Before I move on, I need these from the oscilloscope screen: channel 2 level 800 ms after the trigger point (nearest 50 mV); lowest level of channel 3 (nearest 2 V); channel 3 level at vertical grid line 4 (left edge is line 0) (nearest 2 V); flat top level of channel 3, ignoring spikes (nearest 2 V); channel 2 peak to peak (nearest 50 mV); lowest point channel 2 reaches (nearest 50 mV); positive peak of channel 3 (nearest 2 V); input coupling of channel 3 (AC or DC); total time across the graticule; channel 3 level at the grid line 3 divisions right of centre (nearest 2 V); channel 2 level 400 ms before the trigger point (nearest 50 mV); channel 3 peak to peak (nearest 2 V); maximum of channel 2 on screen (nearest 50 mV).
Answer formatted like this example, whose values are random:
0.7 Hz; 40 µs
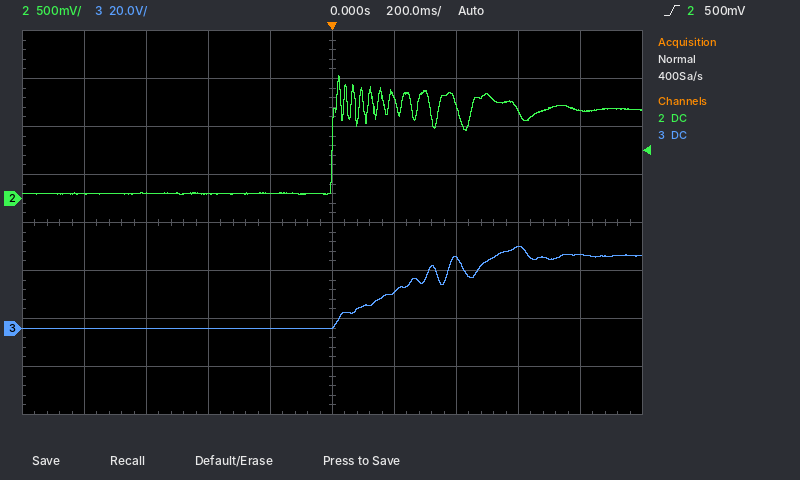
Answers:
900 mV; 0 V; 0 V; 30 V; 1.25 V; 50 mV; 34 V; DC; 2 s; 34 V; 50 mV; 34 V; 1.30 V
